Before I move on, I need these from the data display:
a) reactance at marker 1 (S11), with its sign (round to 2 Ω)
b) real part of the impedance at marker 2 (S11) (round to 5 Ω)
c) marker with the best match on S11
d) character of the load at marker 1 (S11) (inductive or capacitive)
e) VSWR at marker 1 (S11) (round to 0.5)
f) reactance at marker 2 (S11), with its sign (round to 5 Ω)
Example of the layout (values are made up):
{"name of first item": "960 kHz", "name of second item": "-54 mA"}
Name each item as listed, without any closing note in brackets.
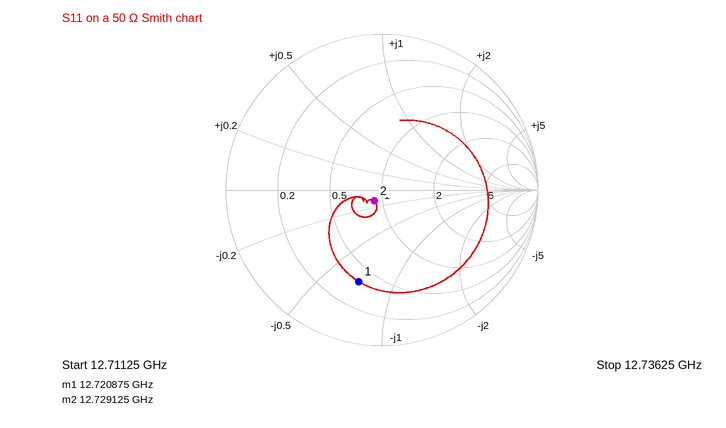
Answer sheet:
{"reactance at marker 1 (S11), with its sign": "-36 Ω", "real part of the impedance at marker 2 (S11)": "45 Ω", "marker with the best match on S11": "marker 2", "character of the load at marker 1 (S11)": "capacitive", "VSWR at marker 1 (S11)": "4.0", "reactance at marker 2 (S11), with its sign": "-5 Ω"}
